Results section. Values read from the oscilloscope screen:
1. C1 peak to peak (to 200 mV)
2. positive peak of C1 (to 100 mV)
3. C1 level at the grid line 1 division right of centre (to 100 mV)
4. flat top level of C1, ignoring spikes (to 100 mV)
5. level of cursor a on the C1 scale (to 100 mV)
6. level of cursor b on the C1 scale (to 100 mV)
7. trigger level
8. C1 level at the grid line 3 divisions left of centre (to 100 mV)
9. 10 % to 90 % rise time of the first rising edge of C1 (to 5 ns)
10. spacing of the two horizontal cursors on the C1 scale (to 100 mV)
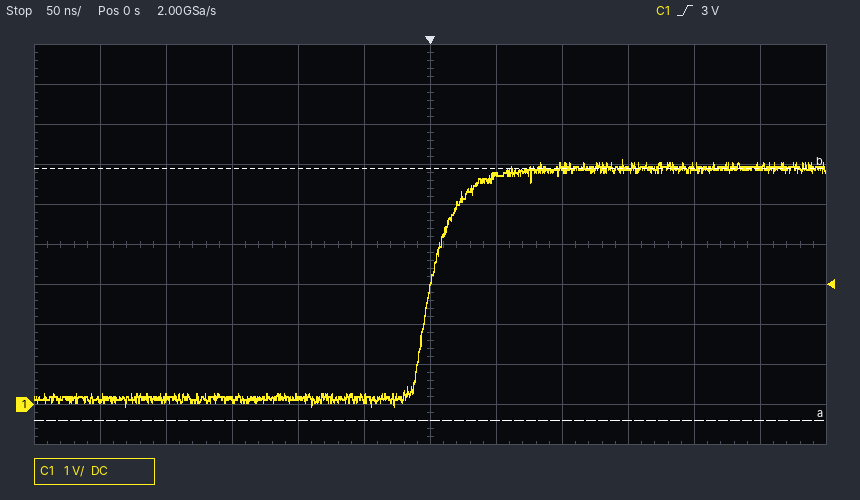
6.2 V
6.1 V
5.7 V
5.9 V
-400 mV
5.9 V
3 V
100 mV
40 ns
6.3 V
